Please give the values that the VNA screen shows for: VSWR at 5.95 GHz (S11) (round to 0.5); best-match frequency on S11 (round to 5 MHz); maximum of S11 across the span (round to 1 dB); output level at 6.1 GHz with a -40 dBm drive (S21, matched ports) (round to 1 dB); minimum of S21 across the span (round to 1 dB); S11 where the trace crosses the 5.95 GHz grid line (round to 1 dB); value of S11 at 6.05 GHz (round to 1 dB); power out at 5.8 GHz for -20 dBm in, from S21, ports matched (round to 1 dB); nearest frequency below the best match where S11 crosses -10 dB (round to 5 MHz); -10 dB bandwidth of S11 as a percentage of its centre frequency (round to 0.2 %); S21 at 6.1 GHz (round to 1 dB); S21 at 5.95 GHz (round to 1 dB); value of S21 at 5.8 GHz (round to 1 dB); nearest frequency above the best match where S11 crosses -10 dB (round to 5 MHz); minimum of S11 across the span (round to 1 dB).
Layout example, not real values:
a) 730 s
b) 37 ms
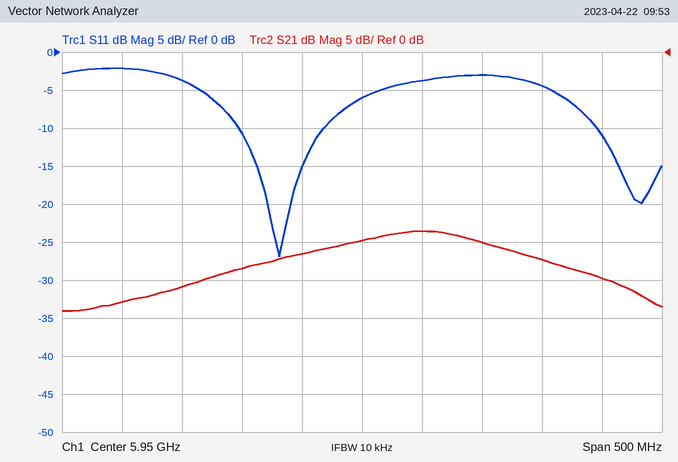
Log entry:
a) 3.0
b) 5.880 GHz
c) -2 dB
d) -67 dBm
e) -34 dB
f) -6 dB
g) -3 dB
h) -51 dBm
i) 5.845 GHz
j) 1.2 %
k) -27 dB
l) -25 dB
m) -31 dB
n) 5.920 GHz
o) -27 dB
